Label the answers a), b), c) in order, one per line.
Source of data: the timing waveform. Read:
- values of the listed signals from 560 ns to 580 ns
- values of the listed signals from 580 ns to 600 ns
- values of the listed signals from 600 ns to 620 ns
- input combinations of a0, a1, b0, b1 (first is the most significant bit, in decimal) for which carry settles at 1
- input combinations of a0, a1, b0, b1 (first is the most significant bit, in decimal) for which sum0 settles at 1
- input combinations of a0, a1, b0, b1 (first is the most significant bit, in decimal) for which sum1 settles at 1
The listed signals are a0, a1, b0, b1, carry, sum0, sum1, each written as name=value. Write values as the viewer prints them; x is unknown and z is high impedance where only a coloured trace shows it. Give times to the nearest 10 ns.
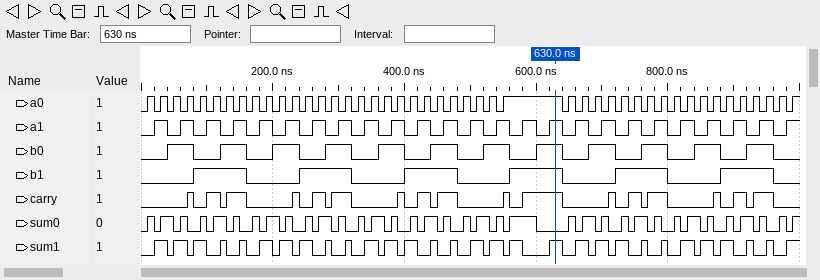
a) a0=1, a1=0, b0=0, b1=1, carry=0, sum0=1, sum1=1
b) a0=1, a1=1, b0=0, b1=1, carry=1, sum0=1, sum1=0
c) a0=1, a1=0, b0=1, b1=1, carry=1, sum0=0, sum1=0
d) 5, 7, 11, 13, 14, 15
e) 2, 3, 6, 7, 8, 9, 12, 13
f) 1, 3, 4, 6, 9, 10, 12, 15
